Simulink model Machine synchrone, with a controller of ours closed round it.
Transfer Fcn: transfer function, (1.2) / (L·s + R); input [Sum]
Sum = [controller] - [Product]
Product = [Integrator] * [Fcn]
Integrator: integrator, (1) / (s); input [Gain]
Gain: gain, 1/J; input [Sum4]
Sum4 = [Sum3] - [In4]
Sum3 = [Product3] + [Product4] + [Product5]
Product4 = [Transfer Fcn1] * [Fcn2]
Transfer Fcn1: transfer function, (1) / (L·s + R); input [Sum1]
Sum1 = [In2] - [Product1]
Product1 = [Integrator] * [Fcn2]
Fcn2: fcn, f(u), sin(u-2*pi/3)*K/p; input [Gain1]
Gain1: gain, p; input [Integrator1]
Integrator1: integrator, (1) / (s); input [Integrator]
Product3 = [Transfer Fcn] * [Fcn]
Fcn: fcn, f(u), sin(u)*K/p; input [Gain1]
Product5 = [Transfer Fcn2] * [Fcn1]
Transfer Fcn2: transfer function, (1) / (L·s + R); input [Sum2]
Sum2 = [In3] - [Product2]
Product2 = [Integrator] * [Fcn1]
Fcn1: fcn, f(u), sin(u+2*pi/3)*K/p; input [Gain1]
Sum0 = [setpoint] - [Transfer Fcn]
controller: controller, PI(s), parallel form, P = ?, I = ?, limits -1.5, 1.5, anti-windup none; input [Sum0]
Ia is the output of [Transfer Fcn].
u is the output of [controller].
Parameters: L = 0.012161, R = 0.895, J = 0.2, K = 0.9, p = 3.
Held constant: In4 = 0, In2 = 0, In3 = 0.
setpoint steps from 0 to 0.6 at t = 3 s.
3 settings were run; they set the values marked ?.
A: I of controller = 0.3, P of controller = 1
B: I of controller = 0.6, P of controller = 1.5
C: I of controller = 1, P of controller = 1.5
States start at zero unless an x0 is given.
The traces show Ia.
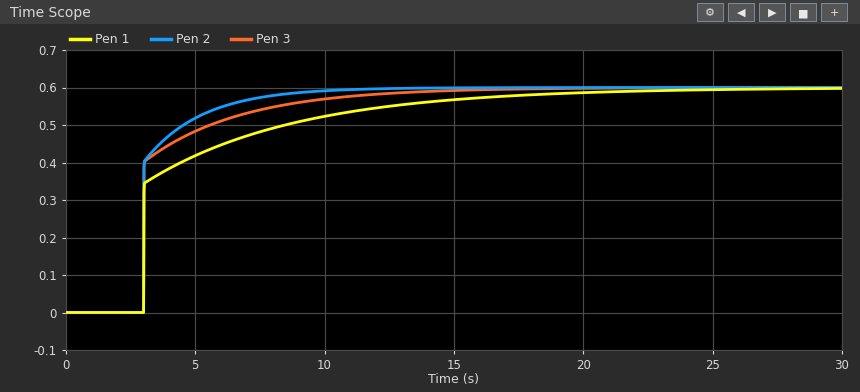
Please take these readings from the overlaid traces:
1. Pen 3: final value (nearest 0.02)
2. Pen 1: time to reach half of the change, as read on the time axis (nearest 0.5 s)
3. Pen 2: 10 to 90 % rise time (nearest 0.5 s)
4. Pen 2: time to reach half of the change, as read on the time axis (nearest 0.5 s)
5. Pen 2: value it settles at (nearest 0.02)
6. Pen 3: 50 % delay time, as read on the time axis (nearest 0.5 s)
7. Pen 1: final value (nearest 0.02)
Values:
0.60
3.0 s
2.5 s
3.0 s
0.60
3.0 s
0.60
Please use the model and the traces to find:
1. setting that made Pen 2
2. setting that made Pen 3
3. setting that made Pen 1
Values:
C
B
A
